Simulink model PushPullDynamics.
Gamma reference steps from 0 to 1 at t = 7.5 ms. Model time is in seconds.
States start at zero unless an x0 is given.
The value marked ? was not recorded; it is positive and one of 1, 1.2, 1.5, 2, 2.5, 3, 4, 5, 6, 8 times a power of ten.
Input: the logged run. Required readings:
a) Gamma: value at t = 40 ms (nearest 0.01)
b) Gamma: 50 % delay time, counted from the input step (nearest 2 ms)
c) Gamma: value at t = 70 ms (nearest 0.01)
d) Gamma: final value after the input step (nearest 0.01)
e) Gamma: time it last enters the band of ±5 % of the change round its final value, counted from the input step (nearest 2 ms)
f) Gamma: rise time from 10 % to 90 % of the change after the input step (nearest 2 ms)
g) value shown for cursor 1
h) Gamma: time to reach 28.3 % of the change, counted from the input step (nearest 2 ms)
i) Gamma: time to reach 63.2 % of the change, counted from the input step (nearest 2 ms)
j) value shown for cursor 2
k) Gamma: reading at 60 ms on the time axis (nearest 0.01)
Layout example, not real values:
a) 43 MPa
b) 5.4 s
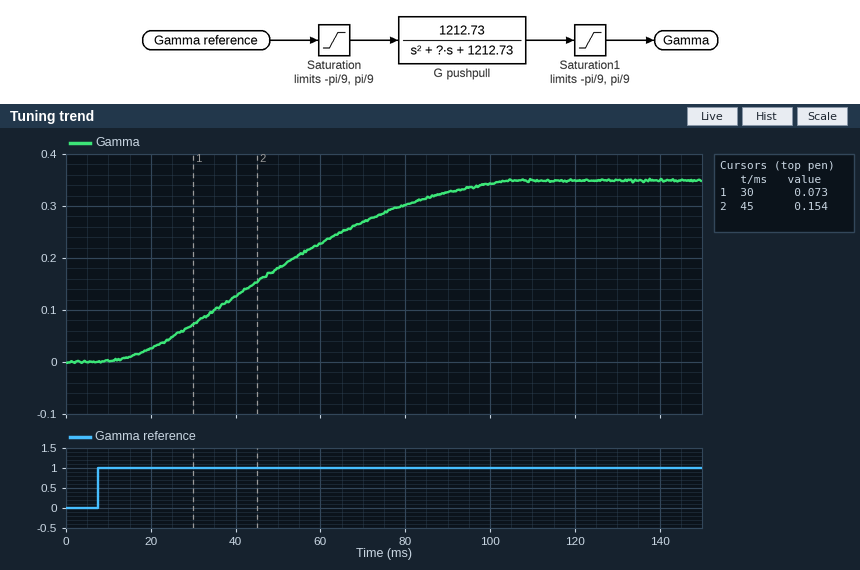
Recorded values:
a) 0.13
b) 42 ms
c) 0.27
d) 0.35
e) 86 ms
f) 62 ms
g) 0.073
h) 28 ms
i) 50 ms
j) 0.154
k) 0.23
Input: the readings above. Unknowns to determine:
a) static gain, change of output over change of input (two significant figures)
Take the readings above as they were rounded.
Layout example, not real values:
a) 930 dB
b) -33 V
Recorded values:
a) 0.35
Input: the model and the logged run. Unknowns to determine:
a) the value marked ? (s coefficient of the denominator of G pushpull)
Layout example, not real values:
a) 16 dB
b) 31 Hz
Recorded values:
a) 50
